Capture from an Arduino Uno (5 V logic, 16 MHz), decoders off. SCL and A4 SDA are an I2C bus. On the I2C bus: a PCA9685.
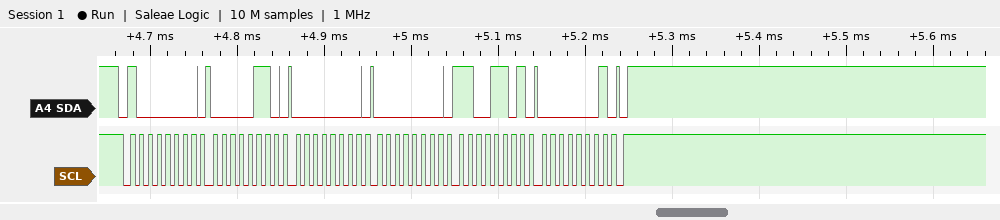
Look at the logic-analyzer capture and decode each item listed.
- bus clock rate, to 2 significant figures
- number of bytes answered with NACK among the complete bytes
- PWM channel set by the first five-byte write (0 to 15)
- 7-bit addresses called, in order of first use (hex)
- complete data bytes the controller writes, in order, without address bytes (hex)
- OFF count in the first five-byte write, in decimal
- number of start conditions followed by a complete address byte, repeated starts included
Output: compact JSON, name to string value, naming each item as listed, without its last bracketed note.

{"bus clock rate, to 2 significant figures": "100 kHz", "number of bytes answered with NACK among the complete bytes": "0", "PWM channel set by the first five-byte write": "0", "7-bit addresses called, in order of first use": "0x40", "complete data bytes the controller writes, in order, without address bytes": "06 00 00 CD 01", "OFF count in the first five-byte write, in decimal": "461", "number of start conditions followed by a complete address byte, repeated starts included": "1"}
